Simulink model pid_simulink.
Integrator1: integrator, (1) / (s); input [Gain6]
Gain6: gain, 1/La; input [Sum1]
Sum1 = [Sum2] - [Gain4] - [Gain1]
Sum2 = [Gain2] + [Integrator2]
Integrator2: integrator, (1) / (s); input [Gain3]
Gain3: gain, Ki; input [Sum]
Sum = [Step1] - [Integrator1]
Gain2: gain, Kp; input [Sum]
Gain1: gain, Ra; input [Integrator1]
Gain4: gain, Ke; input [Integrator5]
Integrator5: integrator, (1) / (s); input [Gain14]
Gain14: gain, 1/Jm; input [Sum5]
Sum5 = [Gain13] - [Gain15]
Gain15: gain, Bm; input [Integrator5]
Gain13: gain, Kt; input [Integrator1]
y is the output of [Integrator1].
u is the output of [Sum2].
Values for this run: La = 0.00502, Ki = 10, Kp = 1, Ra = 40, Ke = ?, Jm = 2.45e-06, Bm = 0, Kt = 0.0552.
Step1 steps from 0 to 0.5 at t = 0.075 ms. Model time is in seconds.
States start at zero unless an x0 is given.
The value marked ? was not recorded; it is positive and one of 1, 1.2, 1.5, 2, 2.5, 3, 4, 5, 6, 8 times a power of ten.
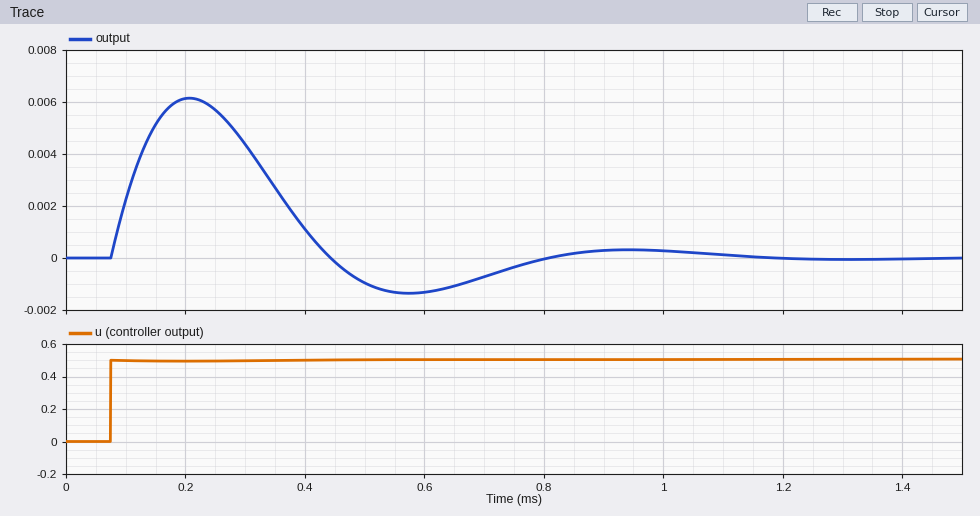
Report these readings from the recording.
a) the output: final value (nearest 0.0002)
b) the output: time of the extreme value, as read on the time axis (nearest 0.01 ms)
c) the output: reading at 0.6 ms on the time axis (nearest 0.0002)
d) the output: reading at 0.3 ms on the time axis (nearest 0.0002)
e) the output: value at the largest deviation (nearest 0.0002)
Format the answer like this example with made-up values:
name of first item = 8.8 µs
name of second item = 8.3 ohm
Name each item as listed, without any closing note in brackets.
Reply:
the output: final value = 0.0000
the output: time of the extreme value, as read on the time axis = 0.21 ms
the output: reading at 0.6 ms on the time axis = -0.0014
the output: reading at 0.3 ms on the time axis = 0.0044
the output: value at the largest deviation = 0.0062
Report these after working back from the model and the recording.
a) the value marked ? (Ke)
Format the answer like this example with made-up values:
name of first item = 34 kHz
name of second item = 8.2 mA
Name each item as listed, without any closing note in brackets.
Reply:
the value marked ? = 20
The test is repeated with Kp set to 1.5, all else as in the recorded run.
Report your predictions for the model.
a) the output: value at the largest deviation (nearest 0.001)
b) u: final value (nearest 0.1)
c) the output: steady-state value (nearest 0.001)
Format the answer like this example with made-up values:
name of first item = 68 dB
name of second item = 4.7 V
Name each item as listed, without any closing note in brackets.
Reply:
the output: value at the largest deviation = 0.009
u: final value = 0.8
the output: steady-state value = 0.000
